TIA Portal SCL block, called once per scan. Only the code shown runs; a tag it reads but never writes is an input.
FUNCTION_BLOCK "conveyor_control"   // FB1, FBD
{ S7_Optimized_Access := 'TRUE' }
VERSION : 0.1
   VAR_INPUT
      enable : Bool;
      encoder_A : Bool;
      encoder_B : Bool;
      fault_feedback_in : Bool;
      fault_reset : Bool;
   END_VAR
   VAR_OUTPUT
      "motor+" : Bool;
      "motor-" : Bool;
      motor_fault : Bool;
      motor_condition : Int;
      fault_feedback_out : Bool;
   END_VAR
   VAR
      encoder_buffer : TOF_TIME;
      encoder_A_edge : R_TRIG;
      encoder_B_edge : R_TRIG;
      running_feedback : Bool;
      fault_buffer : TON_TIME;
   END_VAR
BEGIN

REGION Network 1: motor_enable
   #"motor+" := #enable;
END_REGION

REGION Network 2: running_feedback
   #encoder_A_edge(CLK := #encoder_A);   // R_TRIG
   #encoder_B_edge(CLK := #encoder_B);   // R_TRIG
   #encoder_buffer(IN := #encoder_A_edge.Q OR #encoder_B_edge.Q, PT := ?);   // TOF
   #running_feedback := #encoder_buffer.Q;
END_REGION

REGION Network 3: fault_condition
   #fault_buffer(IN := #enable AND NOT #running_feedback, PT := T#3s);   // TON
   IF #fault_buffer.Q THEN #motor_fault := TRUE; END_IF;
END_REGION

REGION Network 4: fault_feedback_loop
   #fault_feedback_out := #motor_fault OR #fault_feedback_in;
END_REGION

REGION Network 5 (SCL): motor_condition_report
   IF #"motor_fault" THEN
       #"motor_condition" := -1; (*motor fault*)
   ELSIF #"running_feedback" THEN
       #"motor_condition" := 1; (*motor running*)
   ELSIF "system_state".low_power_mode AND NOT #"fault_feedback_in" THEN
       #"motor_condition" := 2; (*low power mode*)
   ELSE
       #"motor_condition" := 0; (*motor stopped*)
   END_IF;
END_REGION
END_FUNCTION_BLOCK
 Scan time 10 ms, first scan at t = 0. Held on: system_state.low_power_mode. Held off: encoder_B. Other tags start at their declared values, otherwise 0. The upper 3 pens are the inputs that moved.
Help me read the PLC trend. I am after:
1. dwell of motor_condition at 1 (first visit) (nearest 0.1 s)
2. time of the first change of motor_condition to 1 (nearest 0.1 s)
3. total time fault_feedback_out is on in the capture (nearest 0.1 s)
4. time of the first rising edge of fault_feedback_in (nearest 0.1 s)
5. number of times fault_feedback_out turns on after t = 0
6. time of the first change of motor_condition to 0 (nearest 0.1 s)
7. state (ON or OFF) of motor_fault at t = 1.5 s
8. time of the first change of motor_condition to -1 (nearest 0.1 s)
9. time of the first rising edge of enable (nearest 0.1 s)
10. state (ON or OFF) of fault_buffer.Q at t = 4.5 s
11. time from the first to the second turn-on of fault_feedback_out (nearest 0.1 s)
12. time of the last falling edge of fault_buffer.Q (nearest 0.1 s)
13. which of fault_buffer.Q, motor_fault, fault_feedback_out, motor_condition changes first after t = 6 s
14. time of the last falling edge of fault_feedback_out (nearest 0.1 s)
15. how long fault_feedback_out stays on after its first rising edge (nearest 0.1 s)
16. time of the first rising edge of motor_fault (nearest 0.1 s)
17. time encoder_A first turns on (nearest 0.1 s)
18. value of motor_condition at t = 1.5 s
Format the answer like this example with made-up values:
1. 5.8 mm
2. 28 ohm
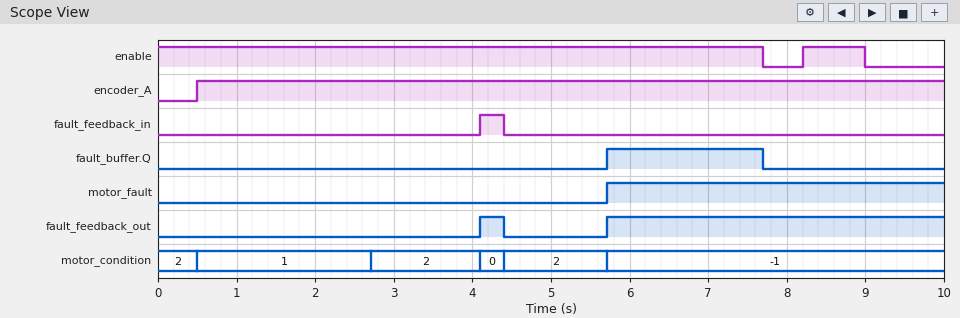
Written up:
1. 2.2 s
2. 0.5 s
3. 4.6 s
4. 4.1 s
5. 2
6. 4.1 s
7. OFF
8. 5.7 s
9. 8.2 s
10. OFF
11. 1.6 s
12. 7.7 s
13. fault_buffer.Q
14. 4.4 s
15. 0.3 s
16. 5.7 s
17. 0.5 s
18. 1
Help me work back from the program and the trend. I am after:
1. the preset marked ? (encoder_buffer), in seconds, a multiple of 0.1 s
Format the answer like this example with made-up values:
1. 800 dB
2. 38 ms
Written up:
1. 2.2 s
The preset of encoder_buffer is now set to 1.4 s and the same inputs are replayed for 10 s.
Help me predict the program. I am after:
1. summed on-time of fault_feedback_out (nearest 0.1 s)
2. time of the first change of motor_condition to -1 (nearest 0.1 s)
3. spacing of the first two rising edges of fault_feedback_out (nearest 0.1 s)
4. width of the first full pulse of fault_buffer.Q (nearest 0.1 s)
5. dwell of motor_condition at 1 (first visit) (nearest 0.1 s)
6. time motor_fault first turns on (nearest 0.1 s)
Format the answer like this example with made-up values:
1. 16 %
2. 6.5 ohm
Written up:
1. 5.4 s
2. 4.9 s
3. 0.8 s
4. 2.8 s
5. 1.4 s
6. 4.9 s
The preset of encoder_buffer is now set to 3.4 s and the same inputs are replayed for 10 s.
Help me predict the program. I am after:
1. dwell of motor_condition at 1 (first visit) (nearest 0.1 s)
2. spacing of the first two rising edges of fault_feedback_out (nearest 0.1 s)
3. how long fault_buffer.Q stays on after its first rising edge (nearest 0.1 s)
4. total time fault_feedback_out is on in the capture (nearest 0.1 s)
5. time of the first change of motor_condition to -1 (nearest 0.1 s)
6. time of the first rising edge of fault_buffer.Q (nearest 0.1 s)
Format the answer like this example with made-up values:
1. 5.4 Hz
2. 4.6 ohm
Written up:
1. 3.4 s
2. 2.8 s
3. 0.8 s
4. 3.4 s
5. 6.9 s
6. 6.9 s
